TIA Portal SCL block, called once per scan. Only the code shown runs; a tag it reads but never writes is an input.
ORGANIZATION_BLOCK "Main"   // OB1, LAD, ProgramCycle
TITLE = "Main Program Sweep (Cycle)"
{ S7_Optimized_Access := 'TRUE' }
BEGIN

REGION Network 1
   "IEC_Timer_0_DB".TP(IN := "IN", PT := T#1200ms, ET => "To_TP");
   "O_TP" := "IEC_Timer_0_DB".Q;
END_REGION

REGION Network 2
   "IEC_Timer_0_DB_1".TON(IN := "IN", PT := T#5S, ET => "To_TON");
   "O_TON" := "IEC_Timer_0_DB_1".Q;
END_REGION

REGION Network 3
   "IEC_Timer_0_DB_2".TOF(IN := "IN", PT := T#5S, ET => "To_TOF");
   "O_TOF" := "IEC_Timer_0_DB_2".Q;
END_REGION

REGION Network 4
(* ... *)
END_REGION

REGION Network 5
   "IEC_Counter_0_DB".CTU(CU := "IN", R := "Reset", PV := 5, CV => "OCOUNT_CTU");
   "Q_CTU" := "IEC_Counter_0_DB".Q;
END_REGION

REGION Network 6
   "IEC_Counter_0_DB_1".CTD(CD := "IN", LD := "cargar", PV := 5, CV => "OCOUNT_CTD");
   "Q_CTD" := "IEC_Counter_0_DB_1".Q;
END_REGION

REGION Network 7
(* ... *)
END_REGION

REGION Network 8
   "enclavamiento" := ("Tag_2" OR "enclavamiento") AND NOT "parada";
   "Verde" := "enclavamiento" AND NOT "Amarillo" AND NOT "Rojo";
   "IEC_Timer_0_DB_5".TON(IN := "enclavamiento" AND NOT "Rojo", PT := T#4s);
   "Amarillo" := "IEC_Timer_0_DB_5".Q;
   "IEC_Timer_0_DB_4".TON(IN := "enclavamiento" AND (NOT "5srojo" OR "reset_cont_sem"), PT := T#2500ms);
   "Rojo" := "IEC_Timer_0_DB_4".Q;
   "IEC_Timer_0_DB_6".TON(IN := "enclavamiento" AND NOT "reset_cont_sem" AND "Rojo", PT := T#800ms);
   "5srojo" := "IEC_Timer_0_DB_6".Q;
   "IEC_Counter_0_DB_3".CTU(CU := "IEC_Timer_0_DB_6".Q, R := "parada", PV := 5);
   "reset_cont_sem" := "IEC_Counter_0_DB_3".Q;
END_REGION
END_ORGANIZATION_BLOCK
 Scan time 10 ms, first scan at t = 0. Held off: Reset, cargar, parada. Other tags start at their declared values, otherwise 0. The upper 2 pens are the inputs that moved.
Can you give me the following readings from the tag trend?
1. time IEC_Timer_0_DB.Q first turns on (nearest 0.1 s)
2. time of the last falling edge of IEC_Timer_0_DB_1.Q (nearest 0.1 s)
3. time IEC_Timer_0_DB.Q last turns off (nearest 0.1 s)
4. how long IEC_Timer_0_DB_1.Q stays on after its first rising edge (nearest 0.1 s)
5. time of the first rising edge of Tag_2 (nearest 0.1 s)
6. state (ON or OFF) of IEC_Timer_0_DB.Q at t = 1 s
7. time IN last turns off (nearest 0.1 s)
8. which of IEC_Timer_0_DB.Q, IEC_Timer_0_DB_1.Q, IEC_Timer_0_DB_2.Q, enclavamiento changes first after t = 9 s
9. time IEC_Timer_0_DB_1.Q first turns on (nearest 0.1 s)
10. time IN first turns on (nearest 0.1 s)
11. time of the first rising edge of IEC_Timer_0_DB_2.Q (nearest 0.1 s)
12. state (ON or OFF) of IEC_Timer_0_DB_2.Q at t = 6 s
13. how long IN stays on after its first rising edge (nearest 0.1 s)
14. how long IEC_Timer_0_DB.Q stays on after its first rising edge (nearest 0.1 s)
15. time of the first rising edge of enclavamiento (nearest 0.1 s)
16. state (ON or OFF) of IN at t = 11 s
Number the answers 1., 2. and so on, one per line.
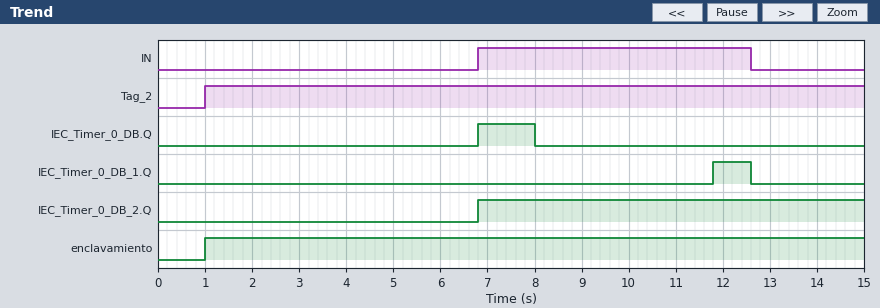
1. 6.8 s
2. 12.6 s
3. 8.0 s
4. 0.8 s
5. 1.0 s
6. OFF
7. 12.6 s
8. IEC_Timer_0_DB_1.Q
9. 11.8 s
10. 6.8 s
11. 6.8 s
12. OFF
13. 5.8 s
14. 1.2 s
15. 1.0 s
16. ON
